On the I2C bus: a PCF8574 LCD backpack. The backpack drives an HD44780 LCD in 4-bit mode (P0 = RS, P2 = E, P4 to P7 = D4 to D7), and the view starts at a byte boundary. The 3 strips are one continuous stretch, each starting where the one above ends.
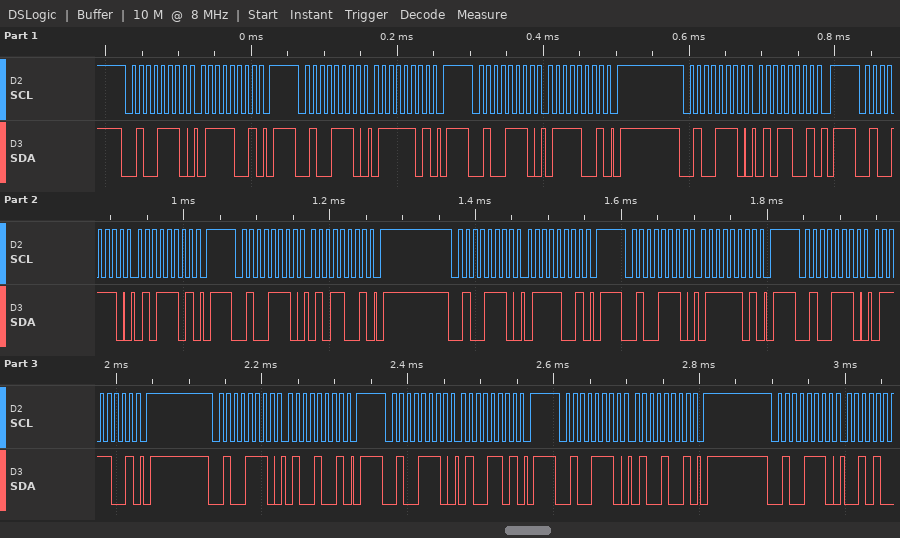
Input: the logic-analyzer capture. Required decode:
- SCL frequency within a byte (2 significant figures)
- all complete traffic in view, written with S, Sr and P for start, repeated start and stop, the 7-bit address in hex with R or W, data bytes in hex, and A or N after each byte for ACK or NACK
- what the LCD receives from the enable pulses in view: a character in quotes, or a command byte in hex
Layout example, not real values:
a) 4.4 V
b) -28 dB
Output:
a) 100 kHz
b) S 27W A 79 A P S 27W A 7D A P S 27W A 79 A P S 27W A 59 A P S 27W A 5D A P S 27W A 59 A P S 27W A 79 A P S 27W A 7D A P S 27W A 79 A P S 27W A 49 A P S 27W A 4D A P S 27W A 49 A P S 27W A
c) 'u' 't'
